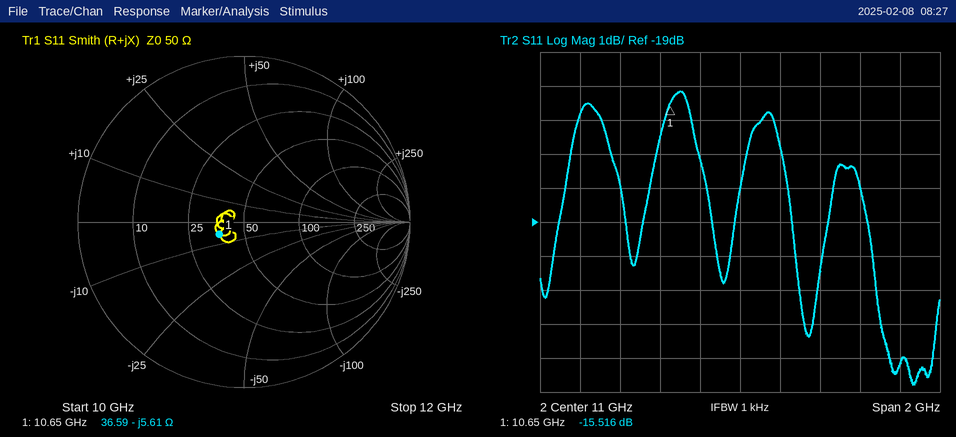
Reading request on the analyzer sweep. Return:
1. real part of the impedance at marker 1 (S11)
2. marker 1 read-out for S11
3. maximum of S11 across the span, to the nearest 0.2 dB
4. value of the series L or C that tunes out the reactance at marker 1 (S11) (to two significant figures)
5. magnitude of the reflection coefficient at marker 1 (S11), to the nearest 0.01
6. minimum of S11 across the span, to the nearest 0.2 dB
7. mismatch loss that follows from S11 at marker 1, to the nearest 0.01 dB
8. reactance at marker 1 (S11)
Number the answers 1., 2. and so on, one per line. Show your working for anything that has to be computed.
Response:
1. 36.59 Ω
2. -15.516 dB
3. -15.2 dB
4. L = 5.61 Ω/(2π × 10.65 GHz) ≈ 84 pH
5. 0.17
6. -23.8 dB
7. −10 log10(1 − 10^(-15.516/10)) ≈ 0.12 dB
8. -5.61 Ω
